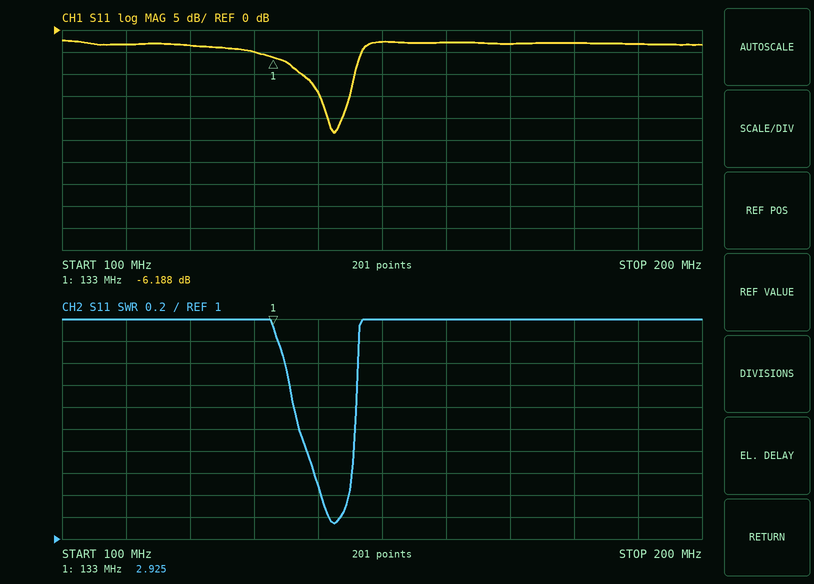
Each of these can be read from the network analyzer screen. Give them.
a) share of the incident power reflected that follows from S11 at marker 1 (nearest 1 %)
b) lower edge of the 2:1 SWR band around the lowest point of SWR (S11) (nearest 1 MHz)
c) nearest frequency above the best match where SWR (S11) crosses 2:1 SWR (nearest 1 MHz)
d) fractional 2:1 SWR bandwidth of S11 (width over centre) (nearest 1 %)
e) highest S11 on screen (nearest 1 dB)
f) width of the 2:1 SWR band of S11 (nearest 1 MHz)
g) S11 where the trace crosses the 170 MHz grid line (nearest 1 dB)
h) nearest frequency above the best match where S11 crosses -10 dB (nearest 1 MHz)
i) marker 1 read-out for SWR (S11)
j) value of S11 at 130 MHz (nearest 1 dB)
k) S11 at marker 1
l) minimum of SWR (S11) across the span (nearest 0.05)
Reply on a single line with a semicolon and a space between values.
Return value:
24 %; 137 MHz; 146 MHz; 6 %; -2 dB; 9 MHz; -3 dB; 146 MHz; 2.925; -5 dB; -6.188 dB; 1.15
